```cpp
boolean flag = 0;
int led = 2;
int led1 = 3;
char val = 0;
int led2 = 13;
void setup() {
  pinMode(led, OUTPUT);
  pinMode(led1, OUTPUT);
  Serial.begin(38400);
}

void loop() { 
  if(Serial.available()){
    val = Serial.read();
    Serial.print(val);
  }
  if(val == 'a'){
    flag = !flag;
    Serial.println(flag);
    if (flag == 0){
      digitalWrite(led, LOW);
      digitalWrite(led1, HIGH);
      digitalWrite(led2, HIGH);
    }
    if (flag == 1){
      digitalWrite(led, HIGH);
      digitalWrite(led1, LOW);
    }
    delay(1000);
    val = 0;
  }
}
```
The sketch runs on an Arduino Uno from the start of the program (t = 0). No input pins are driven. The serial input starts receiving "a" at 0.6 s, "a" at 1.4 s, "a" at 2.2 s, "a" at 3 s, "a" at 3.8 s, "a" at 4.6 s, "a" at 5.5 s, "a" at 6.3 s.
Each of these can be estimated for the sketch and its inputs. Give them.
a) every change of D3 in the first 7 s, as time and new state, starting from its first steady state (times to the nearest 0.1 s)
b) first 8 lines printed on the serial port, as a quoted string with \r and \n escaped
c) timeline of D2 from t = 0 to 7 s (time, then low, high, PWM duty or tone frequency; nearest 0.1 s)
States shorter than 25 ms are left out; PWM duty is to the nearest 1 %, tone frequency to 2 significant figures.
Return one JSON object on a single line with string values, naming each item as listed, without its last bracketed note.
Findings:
{"every change of D3 in the first 7 s, as time and new state, starting from its first steady state": "0 s low; 1.6 s high; 2.6 s low; 3.6 s high; 4.6 s low; 5.6 s high; 6.6 s low", "first 8 lines printed on the serial port, as a quoted string with \\r and \\n escaped": "\"a1\\r\\na0\\r\\na1\\r\\na0\\r\\na1\\r\\na0\\r\\na1\\r\\na0\\r\\n\"", "timeline of D2 from t = 0 to 7 s": "0 s low; 0.6 s high; 1.6 s low; 2.6 s high; 3.6 s low; 4.6 s high; 5.6 s low; 6.6 s high"}
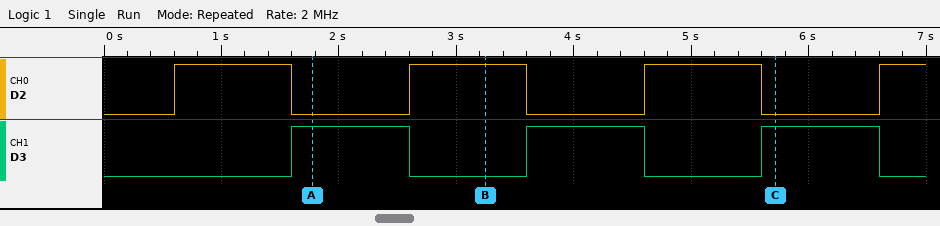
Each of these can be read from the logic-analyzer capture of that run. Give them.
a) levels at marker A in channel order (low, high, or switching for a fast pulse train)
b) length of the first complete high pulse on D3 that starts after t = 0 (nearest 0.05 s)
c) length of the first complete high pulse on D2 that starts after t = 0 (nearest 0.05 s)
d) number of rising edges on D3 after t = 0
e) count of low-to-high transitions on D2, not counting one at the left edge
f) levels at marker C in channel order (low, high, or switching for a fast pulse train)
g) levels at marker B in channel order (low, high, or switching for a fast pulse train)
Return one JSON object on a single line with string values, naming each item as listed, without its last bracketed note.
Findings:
{"levels at marker A in channel order": "D2 low, D3 high", "length of the first complete high pulse on D3 that starts after t = 0": "1.00 s", "length of the first complete high pulse on D2 that starts after t = 0": "1.00 s", "number of rising edges on D3 after t = 0": "3", "count of low-to-high transitions on D2, not counting one at the left edge": "4", "levels at marker C in channel order": "D2 low, D3 high", "levels at marker B in channel order": "D2 high, D3 low"}
